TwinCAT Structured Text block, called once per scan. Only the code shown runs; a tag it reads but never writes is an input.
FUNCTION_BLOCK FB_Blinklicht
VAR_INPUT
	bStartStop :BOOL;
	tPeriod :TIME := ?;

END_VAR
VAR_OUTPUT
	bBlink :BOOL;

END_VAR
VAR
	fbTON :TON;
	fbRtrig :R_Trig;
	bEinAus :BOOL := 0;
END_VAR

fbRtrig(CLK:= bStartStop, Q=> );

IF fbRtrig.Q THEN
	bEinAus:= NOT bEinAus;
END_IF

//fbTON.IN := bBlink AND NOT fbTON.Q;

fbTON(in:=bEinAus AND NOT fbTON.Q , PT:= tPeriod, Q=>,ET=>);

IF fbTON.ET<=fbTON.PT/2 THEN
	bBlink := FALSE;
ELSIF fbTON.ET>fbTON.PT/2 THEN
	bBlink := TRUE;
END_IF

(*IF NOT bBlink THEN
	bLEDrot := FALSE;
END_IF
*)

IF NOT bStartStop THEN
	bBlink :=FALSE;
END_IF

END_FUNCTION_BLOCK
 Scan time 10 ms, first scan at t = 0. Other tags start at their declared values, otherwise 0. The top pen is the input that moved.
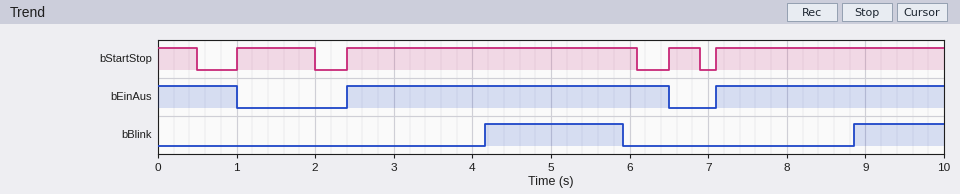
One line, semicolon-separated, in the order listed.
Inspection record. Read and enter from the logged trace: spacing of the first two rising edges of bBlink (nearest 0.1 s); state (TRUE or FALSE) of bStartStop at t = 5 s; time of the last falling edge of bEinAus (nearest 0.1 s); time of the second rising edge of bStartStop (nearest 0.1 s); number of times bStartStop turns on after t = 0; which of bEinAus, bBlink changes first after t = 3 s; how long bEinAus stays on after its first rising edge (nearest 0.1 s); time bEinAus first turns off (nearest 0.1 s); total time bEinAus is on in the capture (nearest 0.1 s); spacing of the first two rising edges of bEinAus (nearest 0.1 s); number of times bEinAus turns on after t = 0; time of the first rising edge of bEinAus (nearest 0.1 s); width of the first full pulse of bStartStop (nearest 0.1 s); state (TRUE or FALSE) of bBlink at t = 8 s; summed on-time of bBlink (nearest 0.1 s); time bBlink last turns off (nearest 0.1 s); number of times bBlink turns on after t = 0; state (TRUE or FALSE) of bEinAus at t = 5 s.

4.7 s; TRUE; 6.5 s; 2.4 s; 4; bBlink; 4.1 s; 1.0 s; 8.0 s; 4.7 s; 2; 2.4 s; 1.0 s; FALSE; 2.9 s; 5.9 s; 2; TRUE
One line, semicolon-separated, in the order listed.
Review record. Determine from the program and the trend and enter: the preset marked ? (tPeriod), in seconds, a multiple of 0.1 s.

3.5 s
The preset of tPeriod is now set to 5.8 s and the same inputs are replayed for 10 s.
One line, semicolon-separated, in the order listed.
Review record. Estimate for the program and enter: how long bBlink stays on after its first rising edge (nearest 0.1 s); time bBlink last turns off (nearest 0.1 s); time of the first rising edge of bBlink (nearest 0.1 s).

0.8 s; 6.1 s; 5.3 s
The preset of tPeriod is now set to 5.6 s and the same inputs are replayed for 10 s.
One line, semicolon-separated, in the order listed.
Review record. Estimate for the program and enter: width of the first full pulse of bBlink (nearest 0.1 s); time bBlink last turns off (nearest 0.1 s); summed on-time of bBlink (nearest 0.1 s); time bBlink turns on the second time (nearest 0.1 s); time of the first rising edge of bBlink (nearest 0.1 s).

0.9 s; 6.1 s; 1.0 s; 9.9 s; 5.2 s
